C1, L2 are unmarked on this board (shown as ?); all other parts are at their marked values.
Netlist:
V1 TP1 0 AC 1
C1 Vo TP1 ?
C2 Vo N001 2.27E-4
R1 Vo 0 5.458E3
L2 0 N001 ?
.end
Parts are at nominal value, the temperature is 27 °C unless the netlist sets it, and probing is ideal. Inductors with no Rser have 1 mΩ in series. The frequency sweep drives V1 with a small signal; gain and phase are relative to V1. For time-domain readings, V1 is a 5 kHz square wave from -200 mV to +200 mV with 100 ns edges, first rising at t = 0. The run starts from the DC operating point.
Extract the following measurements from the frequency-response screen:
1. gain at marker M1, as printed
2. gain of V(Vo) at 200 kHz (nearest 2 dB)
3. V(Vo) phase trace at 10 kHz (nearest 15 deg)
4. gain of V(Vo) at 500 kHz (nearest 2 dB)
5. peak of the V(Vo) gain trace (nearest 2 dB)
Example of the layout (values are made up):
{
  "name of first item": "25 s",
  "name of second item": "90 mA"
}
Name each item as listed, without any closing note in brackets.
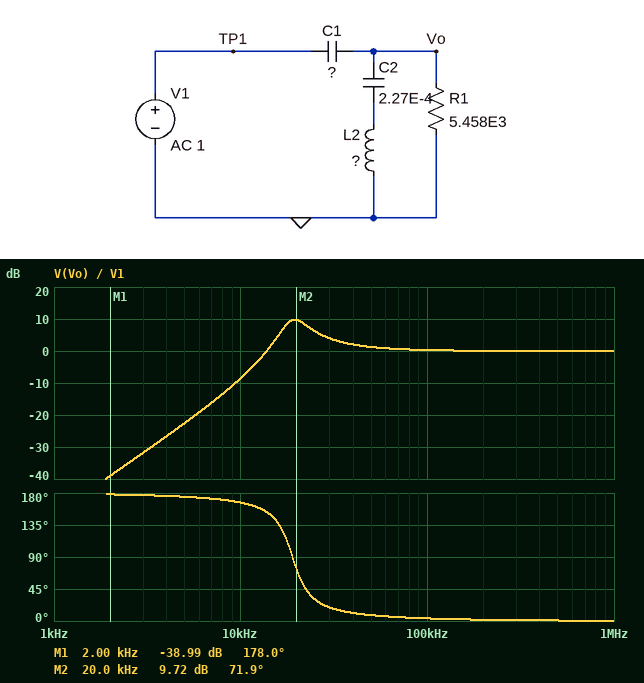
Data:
{
  "gain at marker M1, as printed": "-38.99 dB",
  "gain of V(Vo) at 200 kHz": "0 dB",
  "V(Vo) phase trace at 10 kHz": "165 deg",
  "gain of V(Vo) at 500 kHz": "0 dB",
  "peak of the V(Vo) gain trace": "10 dB"
}
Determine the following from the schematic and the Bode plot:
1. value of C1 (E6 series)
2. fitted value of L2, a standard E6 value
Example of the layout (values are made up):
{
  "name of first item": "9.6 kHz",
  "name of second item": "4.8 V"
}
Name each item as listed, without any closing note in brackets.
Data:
{
  "value of C1": "4.7 nF",
  "fitted value of L2, a standard E6 value": "15 mH"
}
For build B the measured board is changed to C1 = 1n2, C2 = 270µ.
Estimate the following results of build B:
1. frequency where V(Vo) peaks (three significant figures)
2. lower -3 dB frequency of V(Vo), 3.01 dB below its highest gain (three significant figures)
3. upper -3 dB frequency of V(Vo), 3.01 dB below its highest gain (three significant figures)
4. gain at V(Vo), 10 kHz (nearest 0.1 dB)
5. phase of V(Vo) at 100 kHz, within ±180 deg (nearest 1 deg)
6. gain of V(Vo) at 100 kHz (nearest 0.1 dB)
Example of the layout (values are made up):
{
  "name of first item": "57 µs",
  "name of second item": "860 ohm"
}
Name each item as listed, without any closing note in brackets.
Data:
{
  "frequency where V(Vo) peaks": "42.2 kHz",
  "lower -3 dB frequency of V(Vo), 3.01 dB below its highest gain": "31.7 kHz",
  "upper -3 dB frequency of V(Vo), 3.01 dB below its highest gain": "89.1 kHz",
  "gain at V(Vo), 10 kHz": "-22.5 dB",
  "phase of V(Vo) at 100 kHz, within ±180 deg": "16 deg",
  "gain of V(Vo) at 100 kHz": "1.0 dB"
}
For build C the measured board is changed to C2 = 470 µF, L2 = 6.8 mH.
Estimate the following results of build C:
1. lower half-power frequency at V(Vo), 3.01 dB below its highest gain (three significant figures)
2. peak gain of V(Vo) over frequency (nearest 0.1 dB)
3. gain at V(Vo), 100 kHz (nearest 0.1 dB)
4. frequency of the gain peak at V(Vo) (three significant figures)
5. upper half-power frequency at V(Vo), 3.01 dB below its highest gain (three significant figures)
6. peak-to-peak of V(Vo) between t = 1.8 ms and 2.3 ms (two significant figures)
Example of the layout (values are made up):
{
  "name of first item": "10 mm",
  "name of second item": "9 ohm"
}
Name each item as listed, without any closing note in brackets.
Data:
{
  "lower half-power frequency at V(Vo), 3.01 dB below its highest gain": "25.8 kHz",
  "peak gain of V(Vo) over frequency": "13.2 dB",
  "gain at V(Vo), 100 kHz": "0.7 dB",
  "frequency of the gain peak at V(Vo)": "28.5 kHz",
  "upper half-power frequency at V(Vo), 3.01 dB below its highest gain": "32.4 kHz",
  "peak-to-peak of V(Vo) between t = 1.8 ms and 2.3 ms": "740 mV"
}
